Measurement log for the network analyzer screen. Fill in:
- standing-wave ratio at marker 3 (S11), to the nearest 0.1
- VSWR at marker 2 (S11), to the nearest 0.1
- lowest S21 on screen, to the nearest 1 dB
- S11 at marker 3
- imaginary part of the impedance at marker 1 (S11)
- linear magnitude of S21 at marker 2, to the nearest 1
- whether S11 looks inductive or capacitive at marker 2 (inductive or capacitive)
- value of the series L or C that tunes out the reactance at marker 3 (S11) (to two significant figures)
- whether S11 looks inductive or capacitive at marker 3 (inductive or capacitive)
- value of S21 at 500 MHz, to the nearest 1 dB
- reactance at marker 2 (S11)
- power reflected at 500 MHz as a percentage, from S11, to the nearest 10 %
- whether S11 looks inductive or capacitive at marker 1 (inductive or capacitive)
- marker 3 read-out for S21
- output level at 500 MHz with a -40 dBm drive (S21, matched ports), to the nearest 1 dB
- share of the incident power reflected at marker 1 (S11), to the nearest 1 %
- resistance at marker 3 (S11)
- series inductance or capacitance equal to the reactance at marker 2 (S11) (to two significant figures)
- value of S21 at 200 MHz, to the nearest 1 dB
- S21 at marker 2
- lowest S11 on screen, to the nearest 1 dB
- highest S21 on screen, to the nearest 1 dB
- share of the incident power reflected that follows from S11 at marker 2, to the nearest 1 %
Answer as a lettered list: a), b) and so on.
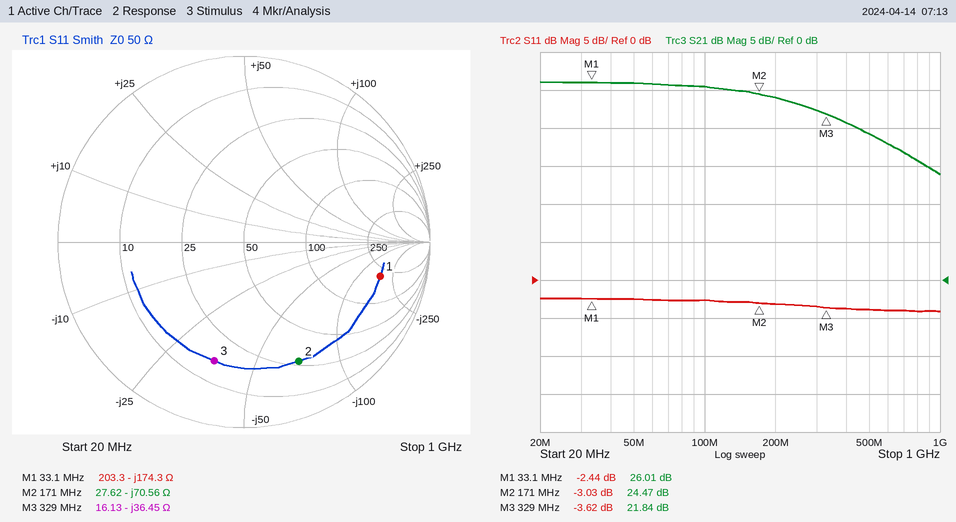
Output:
a) 4.9
b) 5.8
c) 14 dB
d) -3.62 dB
e) -174.3 Ω
f) 17
g) capacitive
h) 18 nH
i) capacitive
j) 19 dB
k) -70.56 Ω
l) 40 %
m) capacitive
n) 21.84 dB
o) -21 dBm
p) 57 %
q) 16.13 Ω
r) 13 pF
s) 24 dB
t) 24.47 dB
u) -4 dB
v) 26 dB
w) 50 %
